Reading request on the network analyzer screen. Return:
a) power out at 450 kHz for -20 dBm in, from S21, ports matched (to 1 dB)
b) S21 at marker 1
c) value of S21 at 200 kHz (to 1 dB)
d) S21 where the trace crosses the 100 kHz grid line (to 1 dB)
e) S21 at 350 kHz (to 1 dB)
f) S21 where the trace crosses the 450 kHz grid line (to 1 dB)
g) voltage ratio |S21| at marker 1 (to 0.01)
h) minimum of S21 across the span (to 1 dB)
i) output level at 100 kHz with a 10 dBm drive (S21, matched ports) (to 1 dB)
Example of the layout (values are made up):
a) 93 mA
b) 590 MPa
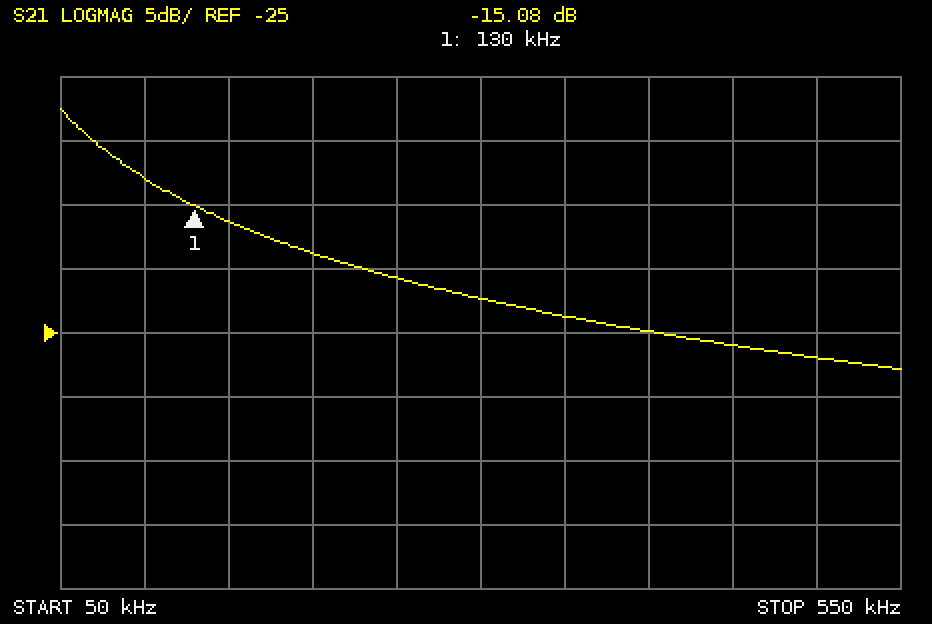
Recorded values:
a) -46 dBm
b) -15.08 dB
c) -19 dB
d) -13 dB
e) -24 dB
f) -26 dB
g) 0.18
h) -28 dB
i) -3 dBm
